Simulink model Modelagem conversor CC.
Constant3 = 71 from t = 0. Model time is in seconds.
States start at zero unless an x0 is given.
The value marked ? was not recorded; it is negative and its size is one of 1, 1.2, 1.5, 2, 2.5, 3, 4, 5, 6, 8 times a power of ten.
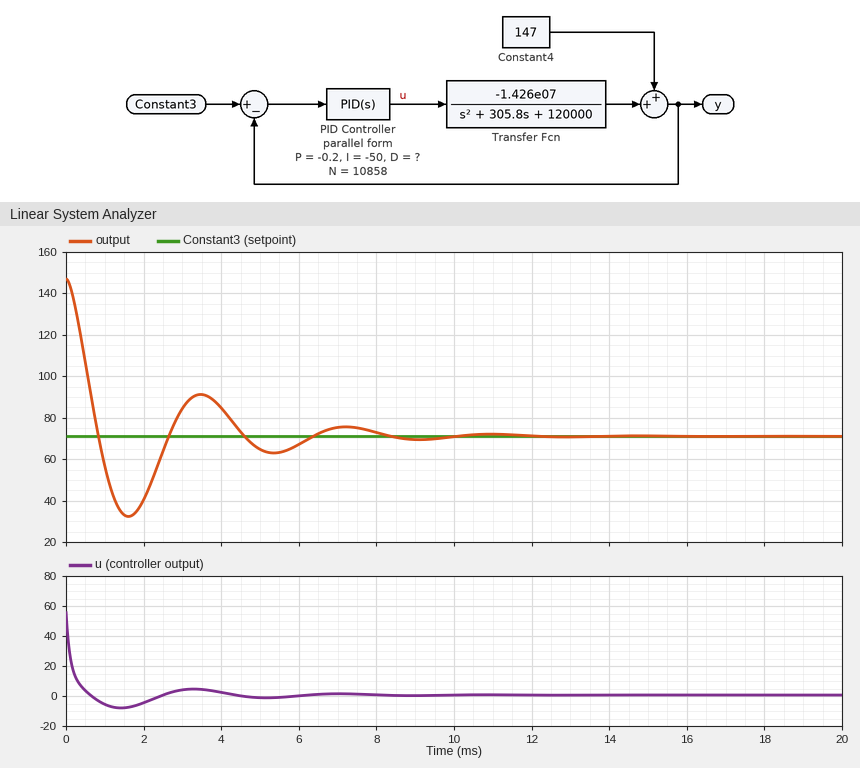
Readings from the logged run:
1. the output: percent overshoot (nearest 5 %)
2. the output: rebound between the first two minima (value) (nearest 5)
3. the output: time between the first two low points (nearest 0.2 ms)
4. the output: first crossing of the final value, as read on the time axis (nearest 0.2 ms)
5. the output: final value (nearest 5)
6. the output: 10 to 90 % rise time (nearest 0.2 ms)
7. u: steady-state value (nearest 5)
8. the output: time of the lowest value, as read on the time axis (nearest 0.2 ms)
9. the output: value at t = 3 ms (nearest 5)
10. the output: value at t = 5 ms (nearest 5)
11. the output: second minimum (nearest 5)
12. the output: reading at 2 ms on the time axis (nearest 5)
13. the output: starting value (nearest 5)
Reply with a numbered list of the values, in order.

1. 50 %
2. 90
3. 3.8 ms
4. 0.8 ms
5. 70
6. 0.6 ms
7. 0
8. 1.6 ms
9. 85
10. 65
11. 65
12. 40
13. 145
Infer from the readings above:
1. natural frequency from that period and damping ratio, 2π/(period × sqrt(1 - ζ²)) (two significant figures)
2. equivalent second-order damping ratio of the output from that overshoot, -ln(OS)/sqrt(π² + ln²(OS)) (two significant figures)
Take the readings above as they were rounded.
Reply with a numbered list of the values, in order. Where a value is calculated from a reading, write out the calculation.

1. 2π / (3.8 × sqrt(1 - 0.22²)) = 1.7 rad/ms
2. ln(0.5) = -0.693; 0.693 / sqrt(9.870 + 0.480) = 0.22
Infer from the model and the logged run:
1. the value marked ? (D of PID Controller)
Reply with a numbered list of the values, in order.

1. -5e-05
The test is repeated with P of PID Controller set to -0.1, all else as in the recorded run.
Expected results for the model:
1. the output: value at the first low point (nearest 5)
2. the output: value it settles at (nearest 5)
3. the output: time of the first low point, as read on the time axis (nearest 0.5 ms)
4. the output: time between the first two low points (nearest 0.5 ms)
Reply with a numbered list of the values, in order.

1. 35
2. 70
3. 2.0 ms
4. 5.5 ms
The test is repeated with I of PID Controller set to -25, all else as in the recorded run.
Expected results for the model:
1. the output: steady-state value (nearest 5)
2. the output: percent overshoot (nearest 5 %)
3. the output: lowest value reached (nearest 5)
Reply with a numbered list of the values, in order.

1. 70
2. 45 %
3. 35
